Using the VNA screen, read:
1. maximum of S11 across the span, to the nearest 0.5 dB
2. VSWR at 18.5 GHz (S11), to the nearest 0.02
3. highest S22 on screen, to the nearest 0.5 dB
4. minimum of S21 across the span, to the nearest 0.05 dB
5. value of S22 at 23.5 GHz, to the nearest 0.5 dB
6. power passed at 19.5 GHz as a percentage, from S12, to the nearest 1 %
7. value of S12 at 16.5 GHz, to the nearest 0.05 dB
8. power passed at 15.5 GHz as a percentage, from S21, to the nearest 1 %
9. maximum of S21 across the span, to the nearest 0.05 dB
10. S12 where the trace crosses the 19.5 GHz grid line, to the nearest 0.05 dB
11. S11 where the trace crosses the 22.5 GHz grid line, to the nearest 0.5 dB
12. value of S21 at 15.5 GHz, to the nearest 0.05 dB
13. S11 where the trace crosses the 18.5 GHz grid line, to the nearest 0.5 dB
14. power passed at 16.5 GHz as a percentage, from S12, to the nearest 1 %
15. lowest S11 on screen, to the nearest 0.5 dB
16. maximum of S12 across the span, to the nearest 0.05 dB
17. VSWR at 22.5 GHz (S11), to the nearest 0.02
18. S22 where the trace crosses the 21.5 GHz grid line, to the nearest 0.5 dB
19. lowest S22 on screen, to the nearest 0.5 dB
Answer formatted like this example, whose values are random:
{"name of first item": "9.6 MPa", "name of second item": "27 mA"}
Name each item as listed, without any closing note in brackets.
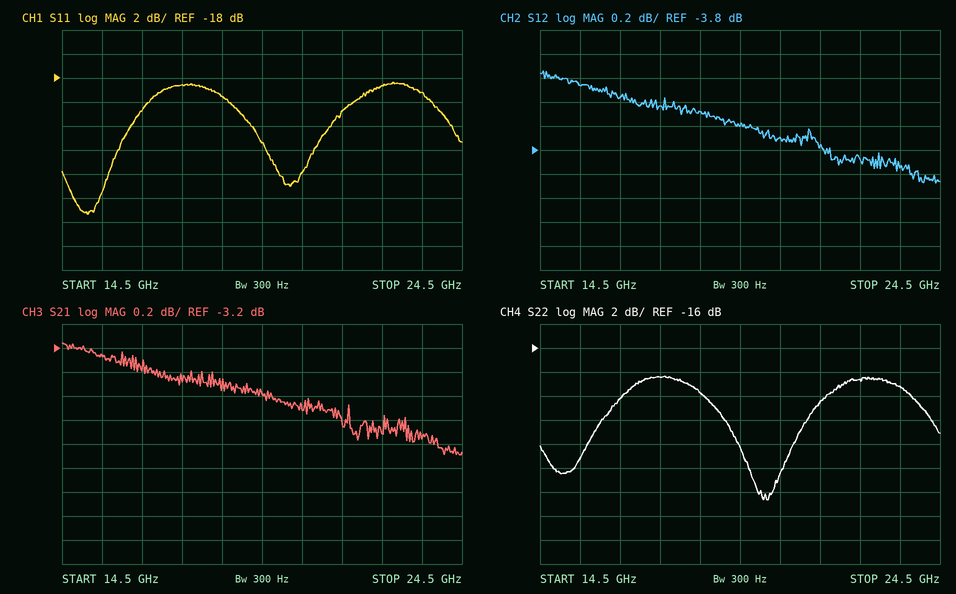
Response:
{"maximum of S11 across the span, to the nearest 0.5 dB": "-18.5 dB", "VSWR at 18.5 GHz (S11), to the nearest 0.02": "1.24", "highest S22 on screen, to the nearest 0.5 dB": "-18.5 dB", "minimum of S21 across the span, to the nearest 0.05 dB": "-4.10 dB", "value of S22 at 23.5 GHz, to the nearest 0.5 dB": "-19.0 dB", "power passed at 19.5 GHz as a percentage, from S12, to the nearest 1 %": "44 %", "value of S12 at 16.5 GHz, to the nearest 0.05 dB": "-3.35 dB", "power passed at 15.5 GHz as a percentage, from S21, to the nearest 1 %": "47 %", "maximum of S21 across the span, to the nearest 0.05 dB": "-3.15 dB", "S12 where the trace crosses the 19.5 GHz grid line, to the nearest 0.05 dB": "-3.60 dB", "S11 where the trace crosses the 22.5 GHz grid line, to the nearest 0.5 dB": "-18.5 dB", "value of S21 at 15.5 GHz, to the nearest 0.05 dB": "-3.25 dB", "S11 where the trace crosses the 18.5 GHz grid line, to the nearest 0.5 dB": "-19.5 dB", "power passed at 16.5 GHz as a percentage, from S12, to the nearest 1 %": "46 %", "lowest S11 on screen, to the nearest 0.5 dB": "-29.5 dB", "maximum of S12 across the span, to the nearest 0.05 dB": "-3.15 dB", "VSWR at 22.5 GHz (S11), to the nearest 0.02": "1.26", "S22 where the trace crosses the 21.5 GHz grid line, to the nearest 0.5 dB": "-20.5 dB", "lowest S22 on screen, to the nearest 0.5 dB": "-28.5 dB"}
